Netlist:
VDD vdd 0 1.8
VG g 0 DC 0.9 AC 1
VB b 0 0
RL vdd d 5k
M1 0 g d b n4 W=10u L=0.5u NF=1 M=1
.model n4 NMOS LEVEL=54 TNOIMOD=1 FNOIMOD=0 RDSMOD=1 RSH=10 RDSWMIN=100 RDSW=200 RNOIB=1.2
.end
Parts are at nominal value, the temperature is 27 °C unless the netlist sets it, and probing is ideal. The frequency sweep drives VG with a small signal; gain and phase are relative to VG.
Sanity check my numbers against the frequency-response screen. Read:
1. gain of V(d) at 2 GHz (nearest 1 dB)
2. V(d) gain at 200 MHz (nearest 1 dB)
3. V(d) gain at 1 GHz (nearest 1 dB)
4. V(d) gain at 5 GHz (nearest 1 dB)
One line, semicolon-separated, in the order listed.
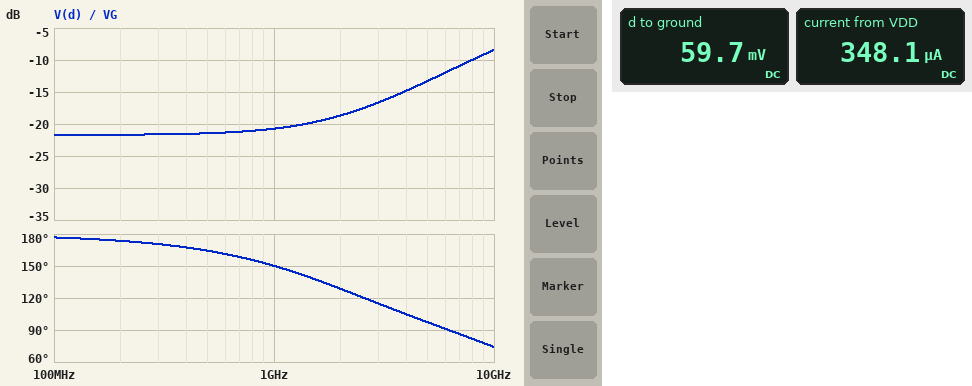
-19 dB; -22 dB; -21 dB; -13 dB
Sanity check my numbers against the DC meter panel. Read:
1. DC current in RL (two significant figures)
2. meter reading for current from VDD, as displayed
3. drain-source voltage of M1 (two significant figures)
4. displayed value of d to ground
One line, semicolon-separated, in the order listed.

350 µA; 348.1 µA; -60 mV; 59.7 mV
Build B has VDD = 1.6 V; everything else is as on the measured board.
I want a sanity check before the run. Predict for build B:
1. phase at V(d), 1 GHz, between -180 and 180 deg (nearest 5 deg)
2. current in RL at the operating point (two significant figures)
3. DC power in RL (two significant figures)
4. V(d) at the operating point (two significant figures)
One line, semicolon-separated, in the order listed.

145 deg; 310 µA; 480 µW; 53 mV
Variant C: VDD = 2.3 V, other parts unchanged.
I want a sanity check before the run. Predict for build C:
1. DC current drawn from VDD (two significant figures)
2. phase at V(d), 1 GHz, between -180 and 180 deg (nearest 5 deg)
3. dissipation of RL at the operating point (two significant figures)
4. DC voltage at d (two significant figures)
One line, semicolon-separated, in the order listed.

440 µA; 155 deg; 990 µW; 78 mV
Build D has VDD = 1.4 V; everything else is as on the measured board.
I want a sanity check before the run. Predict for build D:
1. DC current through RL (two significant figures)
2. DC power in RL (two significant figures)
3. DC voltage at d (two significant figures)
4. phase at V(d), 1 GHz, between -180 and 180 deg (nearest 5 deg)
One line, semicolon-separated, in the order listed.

270 µA; 370 µW; 46 mV; 145 deg
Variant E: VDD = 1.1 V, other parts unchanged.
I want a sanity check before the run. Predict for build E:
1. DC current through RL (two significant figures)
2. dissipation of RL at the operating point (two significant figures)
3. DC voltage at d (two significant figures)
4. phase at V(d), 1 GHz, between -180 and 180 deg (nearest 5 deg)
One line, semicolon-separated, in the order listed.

210 µA; 230 µW; 35 mV; 135 deg
